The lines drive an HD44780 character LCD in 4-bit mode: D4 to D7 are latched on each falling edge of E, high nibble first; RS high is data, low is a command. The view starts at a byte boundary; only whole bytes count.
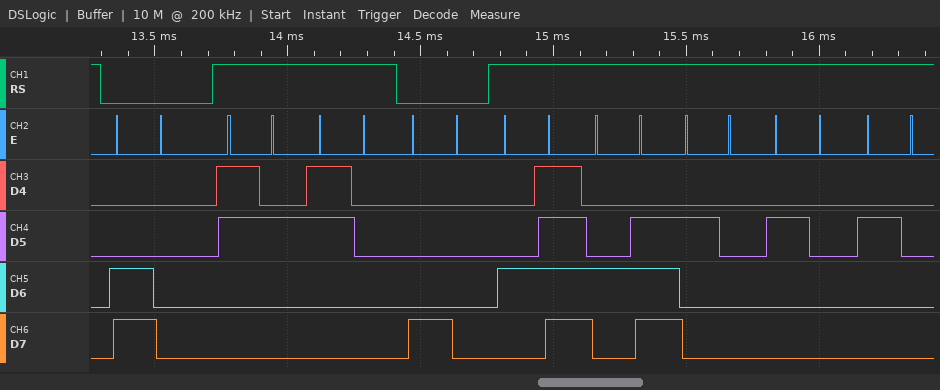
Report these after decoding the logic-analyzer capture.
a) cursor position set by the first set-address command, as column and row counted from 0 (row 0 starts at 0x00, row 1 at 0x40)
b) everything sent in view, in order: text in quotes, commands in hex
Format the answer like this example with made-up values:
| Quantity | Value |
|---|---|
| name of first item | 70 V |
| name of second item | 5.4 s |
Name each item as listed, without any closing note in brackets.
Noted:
| Quantity | Value |
|---|---|
| cursor position set by the first set-address command, as column and row counted from 0 | column 0, row 1 |
| everything sent in view, in order: text in quotes, commands in hex | 0xC0 "20" 0x80 "ON   " |
